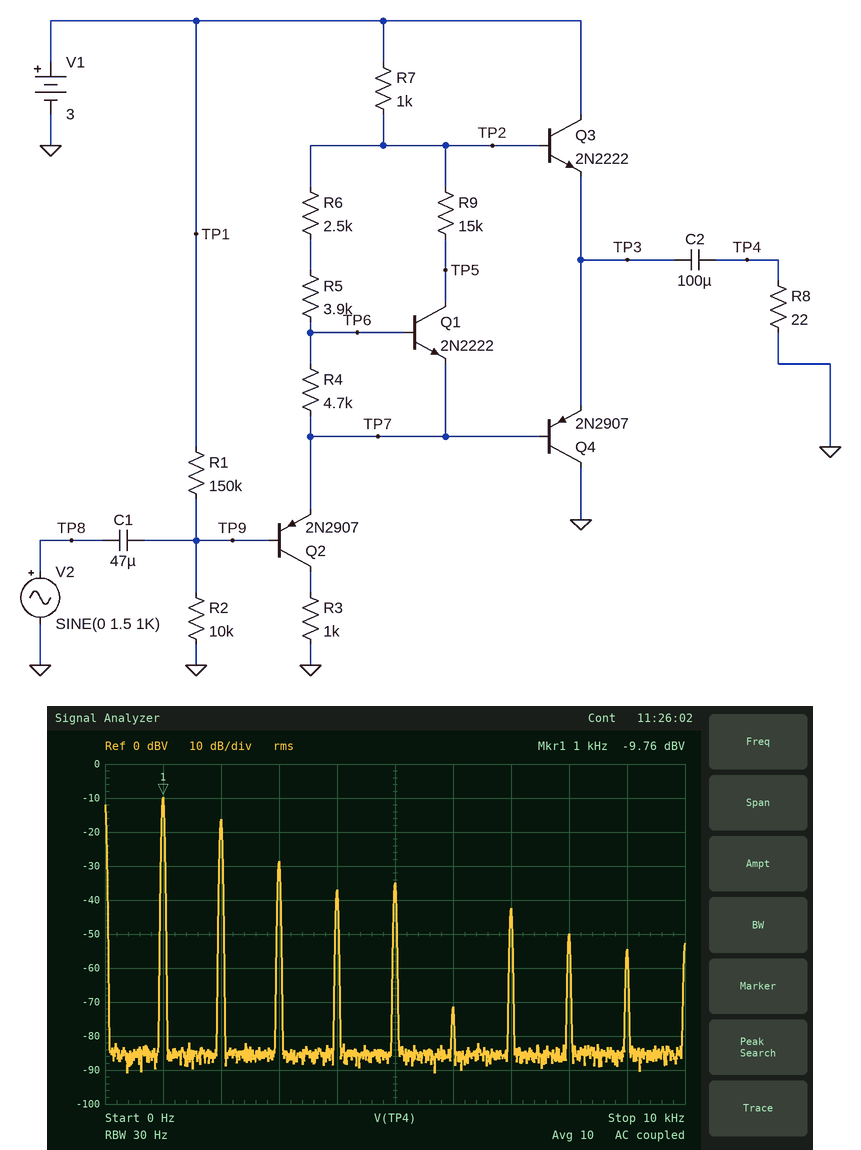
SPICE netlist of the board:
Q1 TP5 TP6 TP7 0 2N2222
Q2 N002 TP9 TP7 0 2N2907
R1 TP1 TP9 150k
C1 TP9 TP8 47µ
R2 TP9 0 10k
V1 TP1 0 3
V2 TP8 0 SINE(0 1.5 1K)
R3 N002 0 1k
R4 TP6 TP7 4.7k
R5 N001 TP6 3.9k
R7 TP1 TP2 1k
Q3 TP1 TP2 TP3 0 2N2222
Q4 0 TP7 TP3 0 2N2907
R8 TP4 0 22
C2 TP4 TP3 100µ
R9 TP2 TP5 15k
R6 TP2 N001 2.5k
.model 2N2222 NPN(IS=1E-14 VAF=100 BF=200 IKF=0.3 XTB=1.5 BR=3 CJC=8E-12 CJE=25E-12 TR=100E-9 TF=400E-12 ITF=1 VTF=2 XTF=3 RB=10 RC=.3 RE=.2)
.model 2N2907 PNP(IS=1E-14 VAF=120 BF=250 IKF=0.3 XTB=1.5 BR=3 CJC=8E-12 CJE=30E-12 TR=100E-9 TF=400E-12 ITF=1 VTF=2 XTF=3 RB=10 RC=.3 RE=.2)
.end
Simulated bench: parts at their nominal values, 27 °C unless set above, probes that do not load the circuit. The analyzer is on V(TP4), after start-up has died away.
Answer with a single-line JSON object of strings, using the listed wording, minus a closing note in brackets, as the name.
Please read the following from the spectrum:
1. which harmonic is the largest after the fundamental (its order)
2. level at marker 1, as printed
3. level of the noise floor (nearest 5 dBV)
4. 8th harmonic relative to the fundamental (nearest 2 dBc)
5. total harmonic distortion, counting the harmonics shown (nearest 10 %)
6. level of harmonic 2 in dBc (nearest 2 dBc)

{"which harmonic is the largest after the fundamental": "2", "level at marker 1, as printed": "-9.76 dBV", "level of the noise floor": "-85 dBV", "8th harmonic relative to the fundamental": "-40 dBc", "total harmonic distortion, counting the harmonics shown": "50 %", "level of harmonic 2 in dBc": "-6 dBc"}
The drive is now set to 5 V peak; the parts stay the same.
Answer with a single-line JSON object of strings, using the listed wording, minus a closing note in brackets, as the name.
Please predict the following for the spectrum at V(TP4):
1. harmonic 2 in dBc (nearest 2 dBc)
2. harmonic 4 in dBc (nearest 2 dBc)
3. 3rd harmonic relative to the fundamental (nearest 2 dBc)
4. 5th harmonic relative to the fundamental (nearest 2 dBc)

{"harmonic 2 in dBc": "-2 dBc", "harmonic 4 in dBc": "-16 dBc", "3rd harmonic relative to the fundamental": "-8 dBc", "5th harmonic relative to the fundamental": "-42 dBc"}
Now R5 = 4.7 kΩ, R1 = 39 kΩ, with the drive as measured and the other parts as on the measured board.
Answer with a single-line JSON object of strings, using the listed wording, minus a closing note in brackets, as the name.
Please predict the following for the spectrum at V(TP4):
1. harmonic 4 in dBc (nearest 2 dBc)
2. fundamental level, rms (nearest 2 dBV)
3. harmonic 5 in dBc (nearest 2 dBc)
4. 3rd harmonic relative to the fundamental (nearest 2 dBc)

{"harmonic 4 in dBc": "-28 dBc", "fundamental level, rms": "-10 dBV", "harmonic 5 in dBc": "-24 dBc", "3rd harmonic relative to the fundamental": "-18 dBc"}
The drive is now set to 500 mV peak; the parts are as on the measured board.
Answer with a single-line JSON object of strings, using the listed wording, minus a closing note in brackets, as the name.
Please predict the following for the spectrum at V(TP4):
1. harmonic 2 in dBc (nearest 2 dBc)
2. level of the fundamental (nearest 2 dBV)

{"harmonic 2 in dBc": "-18 dBc", "level of the fundamental": "-12 dBV"}
